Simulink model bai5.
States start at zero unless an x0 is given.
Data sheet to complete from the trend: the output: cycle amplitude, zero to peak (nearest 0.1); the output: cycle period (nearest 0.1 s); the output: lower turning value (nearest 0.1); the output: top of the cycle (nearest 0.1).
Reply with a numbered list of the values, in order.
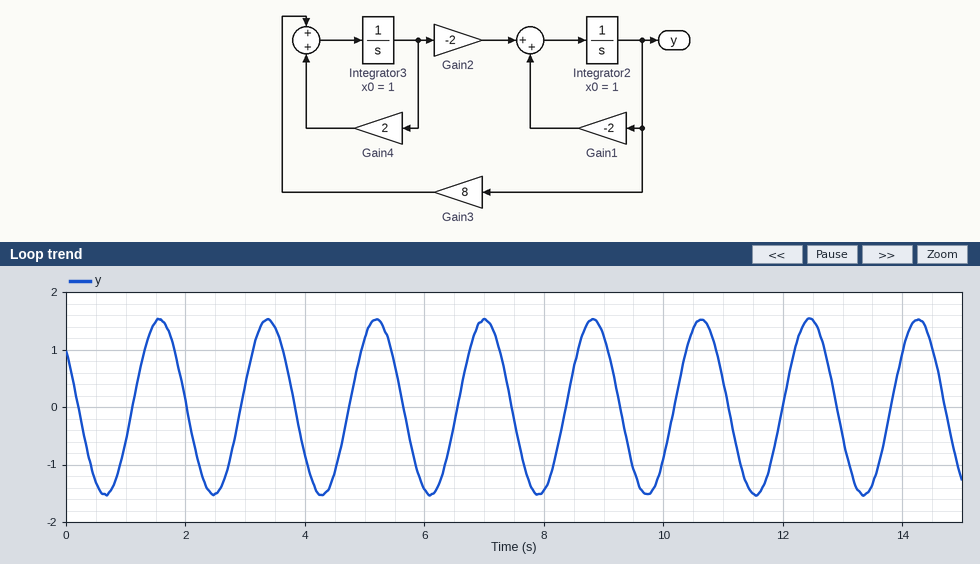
1. 1.5
2. 1.8 s
3. -1.5
4. 1.5
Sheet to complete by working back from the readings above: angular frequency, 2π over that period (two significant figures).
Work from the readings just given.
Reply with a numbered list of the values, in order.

1. 3.5 rad/s
